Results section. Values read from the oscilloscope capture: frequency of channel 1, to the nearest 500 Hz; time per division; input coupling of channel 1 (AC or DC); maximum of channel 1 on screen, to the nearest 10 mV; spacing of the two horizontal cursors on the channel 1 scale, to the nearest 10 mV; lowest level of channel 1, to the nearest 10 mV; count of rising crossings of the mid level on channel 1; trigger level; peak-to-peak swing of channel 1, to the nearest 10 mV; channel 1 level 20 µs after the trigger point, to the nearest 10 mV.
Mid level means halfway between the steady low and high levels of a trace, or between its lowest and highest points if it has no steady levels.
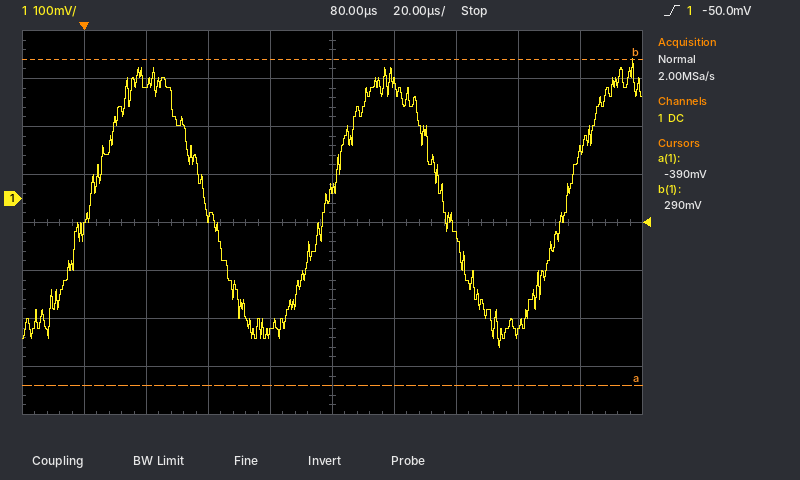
13.0 kHz
20 µs
DC
290 mV
680 mV
-310 mV
3
-50.0 mV
600 mV
240 mV
